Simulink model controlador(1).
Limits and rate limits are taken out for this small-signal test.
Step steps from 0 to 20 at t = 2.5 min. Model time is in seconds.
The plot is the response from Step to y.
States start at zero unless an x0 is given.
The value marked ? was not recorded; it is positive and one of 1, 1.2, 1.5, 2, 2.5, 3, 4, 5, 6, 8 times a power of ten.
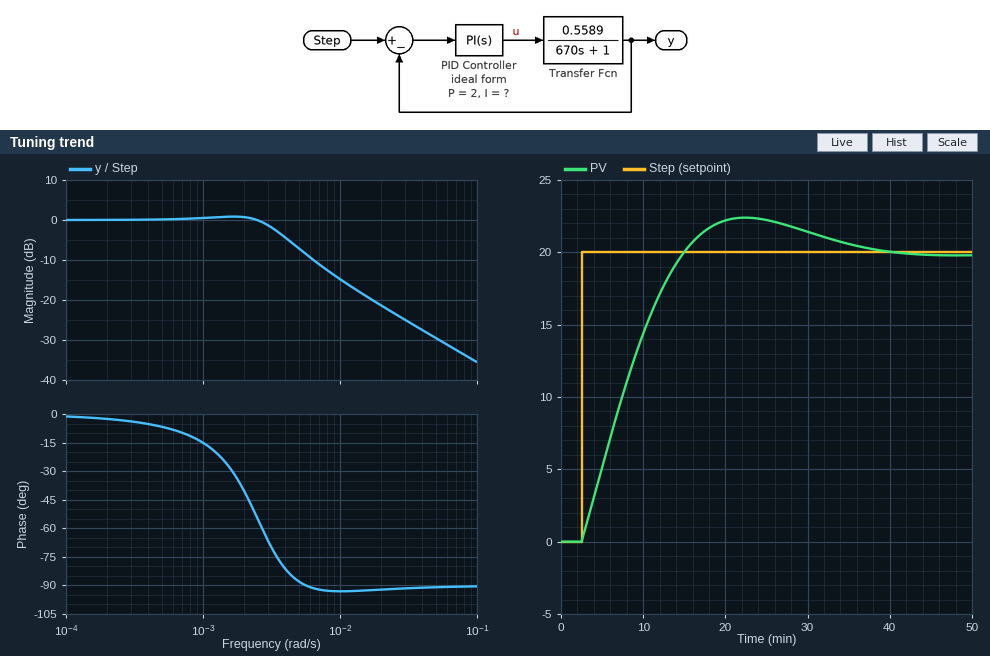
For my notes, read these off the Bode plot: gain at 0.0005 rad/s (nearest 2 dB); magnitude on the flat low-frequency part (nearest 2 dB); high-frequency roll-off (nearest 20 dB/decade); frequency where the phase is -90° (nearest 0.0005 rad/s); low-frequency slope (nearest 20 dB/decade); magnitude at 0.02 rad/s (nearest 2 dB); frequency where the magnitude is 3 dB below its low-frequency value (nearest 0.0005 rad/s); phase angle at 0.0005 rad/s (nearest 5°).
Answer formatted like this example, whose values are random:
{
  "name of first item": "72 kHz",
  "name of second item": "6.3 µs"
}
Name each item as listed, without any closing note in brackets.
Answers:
{
  "gain at 0.0005 rad/s": "0 dB",
  "magnitude on the flat low-frequency part": "0 dB",
  "high-frequency roll-off": "-20 dB/decade",
  "frequency where the phase is -90°": "0.0055 rad/s",
  "low-frequency slope": "0 dB/decade",
  "magnitude at 0.02 rad/s": "-22 dB",
  "frequency where the magnitude is 3 dB below its low-frequency value": "0.0035 rad/s",
  "phase angle at 0.0005 rad/s": "-5°"
}
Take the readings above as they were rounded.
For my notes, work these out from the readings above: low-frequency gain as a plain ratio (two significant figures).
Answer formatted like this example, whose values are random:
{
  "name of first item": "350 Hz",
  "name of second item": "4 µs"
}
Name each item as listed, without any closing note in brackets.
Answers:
{
  "low-frequency gain as a plain ratio": "1.0"
}
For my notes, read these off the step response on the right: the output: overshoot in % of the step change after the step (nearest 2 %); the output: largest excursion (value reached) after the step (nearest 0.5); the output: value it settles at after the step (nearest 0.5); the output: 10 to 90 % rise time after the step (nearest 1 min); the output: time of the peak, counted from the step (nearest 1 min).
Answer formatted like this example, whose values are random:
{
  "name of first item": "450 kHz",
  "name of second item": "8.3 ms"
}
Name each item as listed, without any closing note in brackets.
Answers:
{
  "the output: overshoot in % of the step change after the step": "12 %",
  "the output: largest excursion (value reached) after the step": "22.5",
  "the output: value it settles at after the step": "20.0",
  "the output: 10 to 90 % rise time after the step": "9 min",
  "the output: time of the peak, counted from the step": "20 min"
}
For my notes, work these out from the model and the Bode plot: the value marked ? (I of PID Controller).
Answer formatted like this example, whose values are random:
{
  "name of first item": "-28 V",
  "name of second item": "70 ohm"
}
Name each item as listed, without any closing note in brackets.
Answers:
{
  "the value marked ?": "0.004"
}
